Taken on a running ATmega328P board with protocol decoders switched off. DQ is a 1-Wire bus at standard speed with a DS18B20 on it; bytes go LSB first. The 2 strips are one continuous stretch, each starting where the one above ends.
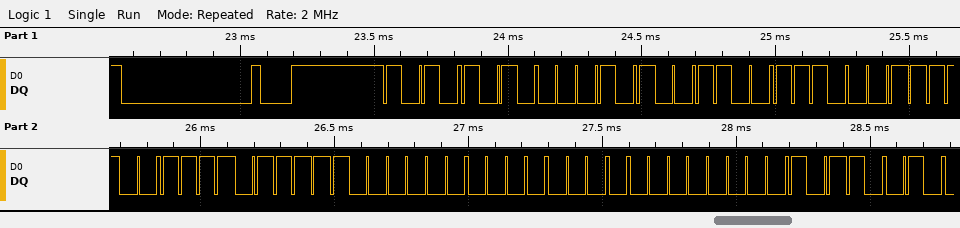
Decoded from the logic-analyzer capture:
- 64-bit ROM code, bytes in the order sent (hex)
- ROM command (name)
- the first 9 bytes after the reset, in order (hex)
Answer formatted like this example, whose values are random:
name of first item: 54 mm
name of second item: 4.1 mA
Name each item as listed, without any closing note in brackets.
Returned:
64-bit ROM code, bytes in the order sent: 28 73 3C EF 03 00 00 4D
ROM command: Match ROM
the first 9 bytes after the reset, in order: 55 28 73 3C EF 03 00 00 4D
